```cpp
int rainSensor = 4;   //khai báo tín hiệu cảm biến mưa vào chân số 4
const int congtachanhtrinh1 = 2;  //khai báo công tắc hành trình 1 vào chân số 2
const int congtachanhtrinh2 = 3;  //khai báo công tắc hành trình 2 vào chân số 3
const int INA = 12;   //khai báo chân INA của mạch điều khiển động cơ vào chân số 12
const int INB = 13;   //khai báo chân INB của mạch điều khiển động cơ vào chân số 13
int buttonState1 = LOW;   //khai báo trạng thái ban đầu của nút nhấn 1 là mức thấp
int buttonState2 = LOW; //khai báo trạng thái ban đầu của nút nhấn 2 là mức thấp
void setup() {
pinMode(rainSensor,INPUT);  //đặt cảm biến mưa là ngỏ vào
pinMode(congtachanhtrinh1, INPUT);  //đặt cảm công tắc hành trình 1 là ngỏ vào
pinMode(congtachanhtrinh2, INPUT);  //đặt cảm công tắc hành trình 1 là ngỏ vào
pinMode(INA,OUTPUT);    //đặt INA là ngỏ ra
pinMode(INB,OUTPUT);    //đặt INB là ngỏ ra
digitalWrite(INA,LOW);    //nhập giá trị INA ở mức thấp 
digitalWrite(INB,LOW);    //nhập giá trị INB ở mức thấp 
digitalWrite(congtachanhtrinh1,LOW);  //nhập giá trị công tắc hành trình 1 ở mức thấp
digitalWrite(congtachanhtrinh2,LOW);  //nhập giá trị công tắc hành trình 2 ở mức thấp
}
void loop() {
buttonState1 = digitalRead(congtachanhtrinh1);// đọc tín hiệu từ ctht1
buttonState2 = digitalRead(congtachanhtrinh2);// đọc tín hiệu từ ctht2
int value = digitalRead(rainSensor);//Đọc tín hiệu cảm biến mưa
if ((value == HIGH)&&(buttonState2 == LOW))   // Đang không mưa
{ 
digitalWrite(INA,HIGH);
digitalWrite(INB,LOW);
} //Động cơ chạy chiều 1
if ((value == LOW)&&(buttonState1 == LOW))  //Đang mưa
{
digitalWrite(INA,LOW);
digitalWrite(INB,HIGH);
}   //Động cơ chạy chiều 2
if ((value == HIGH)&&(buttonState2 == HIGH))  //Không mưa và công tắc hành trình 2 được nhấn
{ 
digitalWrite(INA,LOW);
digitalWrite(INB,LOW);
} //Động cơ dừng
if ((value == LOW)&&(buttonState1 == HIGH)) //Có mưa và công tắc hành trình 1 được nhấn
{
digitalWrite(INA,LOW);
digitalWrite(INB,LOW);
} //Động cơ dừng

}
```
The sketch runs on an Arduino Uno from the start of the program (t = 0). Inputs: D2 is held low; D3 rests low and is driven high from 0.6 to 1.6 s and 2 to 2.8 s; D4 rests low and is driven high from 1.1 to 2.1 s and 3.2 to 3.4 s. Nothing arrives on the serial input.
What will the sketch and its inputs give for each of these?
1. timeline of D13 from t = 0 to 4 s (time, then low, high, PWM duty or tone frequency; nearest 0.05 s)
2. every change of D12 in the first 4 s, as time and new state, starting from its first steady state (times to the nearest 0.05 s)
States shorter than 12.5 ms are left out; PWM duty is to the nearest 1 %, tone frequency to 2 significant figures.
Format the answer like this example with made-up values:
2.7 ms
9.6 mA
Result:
0 s high; 1.1 s low; 2.1 s high; 3.2 s low; 3.4 s high
0 s low; 1.6 s high; 2 s low; 3.2 s high; 3.4 s low
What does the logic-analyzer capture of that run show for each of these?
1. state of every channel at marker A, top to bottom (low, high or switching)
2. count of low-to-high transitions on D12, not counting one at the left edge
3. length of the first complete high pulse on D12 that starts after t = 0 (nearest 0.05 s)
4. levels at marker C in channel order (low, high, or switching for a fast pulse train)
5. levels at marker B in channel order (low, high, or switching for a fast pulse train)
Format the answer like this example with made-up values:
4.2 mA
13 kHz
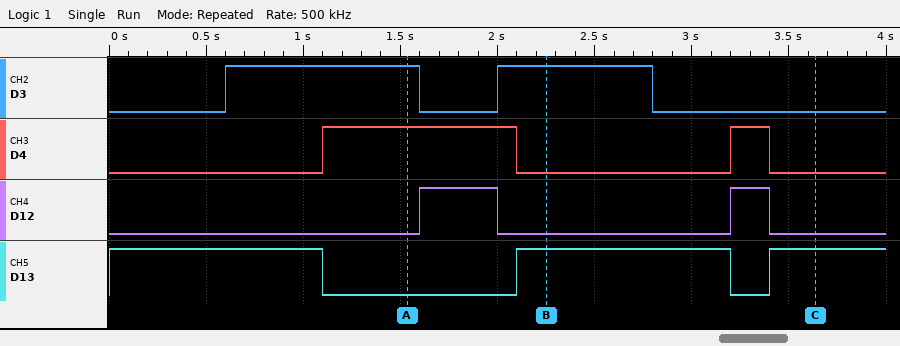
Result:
D3 high, D4 high, D12 low, D13 low
2
0.40 s
D3 low, D4 low, D12 low, D13 high
D3 high, D4 low, D12 low, D13 high
